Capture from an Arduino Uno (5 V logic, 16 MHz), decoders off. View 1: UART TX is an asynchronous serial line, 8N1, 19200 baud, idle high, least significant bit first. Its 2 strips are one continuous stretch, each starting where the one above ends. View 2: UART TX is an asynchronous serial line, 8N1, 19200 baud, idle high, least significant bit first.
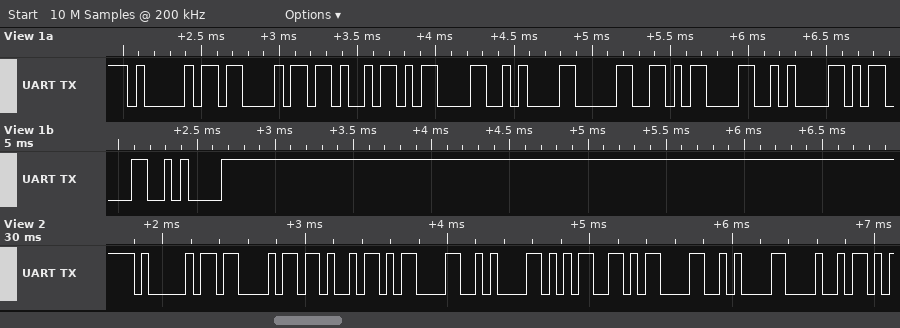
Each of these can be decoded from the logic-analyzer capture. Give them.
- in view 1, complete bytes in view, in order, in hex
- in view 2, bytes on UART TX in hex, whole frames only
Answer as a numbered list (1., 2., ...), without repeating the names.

1. 41 43 4B 0D 0A 30 0D 0A 0D 0A
2. 41 43 4B 0D 0A 35 0D 0A 48
